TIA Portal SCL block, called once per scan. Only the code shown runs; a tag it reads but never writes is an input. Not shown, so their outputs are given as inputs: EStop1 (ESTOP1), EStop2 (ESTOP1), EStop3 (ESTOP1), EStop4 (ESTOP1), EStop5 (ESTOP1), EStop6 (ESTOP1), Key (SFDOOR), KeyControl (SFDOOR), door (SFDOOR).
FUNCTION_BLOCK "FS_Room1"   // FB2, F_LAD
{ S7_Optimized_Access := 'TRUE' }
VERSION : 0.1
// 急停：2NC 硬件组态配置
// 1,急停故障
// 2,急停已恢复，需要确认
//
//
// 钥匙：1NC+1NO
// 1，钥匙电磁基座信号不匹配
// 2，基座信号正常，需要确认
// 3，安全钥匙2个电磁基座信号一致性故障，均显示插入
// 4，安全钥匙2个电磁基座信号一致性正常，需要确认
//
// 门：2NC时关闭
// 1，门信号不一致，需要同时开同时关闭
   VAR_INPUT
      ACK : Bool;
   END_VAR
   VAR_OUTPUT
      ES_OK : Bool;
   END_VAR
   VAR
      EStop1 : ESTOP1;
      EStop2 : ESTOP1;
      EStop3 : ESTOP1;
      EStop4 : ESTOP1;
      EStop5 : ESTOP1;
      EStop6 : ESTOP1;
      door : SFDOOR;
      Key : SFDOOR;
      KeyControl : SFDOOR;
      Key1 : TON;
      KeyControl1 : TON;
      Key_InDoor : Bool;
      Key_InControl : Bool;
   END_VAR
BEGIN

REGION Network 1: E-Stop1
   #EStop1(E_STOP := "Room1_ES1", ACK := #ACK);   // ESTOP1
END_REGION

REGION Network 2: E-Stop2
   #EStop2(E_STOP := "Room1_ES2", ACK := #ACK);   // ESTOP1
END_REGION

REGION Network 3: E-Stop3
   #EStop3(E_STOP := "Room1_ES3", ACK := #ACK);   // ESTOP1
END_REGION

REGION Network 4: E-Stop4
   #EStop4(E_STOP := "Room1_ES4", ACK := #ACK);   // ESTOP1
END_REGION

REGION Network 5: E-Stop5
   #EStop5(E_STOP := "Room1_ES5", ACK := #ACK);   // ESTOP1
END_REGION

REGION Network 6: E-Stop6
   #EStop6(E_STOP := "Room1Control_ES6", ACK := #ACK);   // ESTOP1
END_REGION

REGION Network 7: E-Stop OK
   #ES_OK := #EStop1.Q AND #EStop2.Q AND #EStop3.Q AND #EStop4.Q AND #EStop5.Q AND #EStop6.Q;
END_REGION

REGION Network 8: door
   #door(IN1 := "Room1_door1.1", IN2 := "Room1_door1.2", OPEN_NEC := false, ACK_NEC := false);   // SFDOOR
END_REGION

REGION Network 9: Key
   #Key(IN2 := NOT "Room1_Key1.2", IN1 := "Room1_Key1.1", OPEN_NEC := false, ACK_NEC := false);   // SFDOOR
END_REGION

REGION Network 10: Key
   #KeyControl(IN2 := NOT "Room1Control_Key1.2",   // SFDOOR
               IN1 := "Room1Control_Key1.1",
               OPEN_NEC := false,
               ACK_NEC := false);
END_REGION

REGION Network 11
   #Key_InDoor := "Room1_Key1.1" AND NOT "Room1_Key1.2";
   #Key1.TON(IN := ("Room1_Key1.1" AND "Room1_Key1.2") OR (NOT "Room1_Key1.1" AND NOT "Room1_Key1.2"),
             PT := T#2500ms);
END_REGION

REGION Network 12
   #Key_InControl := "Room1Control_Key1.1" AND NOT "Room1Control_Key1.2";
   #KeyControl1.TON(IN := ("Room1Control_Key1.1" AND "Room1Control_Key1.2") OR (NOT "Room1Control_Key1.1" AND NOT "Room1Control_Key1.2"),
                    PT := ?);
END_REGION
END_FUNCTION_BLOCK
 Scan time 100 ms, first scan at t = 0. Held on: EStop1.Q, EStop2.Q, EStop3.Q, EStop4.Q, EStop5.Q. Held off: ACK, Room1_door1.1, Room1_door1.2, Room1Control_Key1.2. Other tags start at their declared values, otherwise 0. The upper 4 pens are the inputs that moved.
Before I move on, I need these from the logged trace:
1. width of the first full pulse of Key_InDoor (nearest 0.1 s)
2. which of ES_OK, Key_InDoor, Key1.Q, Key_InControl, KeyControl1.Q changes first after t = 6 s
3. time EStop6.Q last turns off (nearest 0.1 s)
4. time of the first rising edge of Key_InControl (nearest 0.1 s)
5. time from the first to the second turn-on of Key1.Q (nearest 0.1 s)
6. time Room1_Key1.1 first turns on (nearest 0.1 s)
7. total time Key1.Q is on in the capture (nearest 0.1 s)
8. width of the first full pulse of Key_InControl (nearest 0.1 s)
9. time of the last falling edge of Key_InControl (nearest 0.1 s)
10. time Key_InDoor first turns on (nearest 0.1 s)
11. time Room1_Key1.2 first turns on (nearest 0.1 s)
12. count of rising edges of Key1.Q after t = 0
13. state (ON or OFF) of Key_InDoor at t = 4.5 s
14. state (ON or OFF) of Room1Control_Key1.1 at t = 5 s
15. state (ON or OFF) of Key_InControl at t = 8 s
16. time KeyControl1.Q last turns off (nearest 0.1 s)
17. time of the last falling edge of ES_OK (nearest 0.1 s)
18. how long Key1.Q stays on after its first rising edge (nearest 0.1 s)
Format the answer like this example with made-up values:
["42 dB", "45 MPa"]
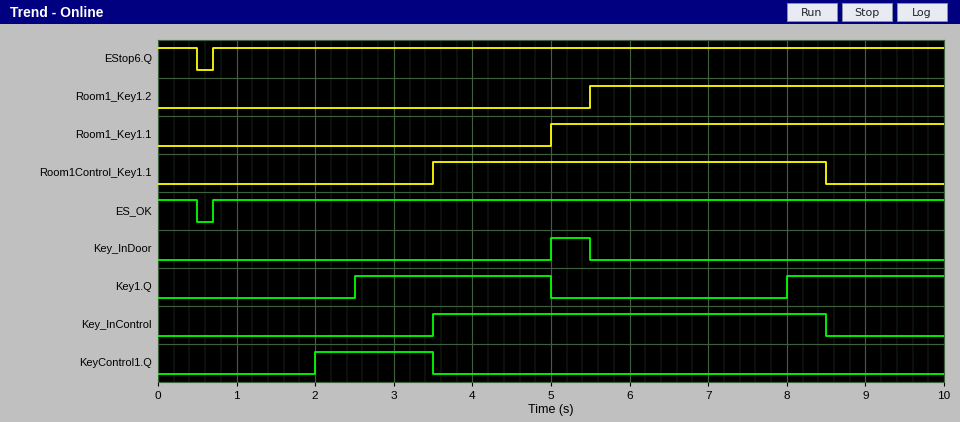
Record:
["0.5 s", "Key1.Q", "0.5 s", "3.5 s", "5.5 s", "5.0 s", "4.5 s", "5.0 s", "8.5 s", "5.0 s", "5.5 s", "2", "OFF", "ON", "ON", "3.5 s", "0.5 s", "2.5 s"]
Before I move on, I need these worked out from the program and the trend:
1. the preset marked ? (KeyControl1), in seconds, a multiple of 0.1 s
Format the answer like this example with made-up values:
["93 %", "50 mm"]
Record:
["2.0 s"]
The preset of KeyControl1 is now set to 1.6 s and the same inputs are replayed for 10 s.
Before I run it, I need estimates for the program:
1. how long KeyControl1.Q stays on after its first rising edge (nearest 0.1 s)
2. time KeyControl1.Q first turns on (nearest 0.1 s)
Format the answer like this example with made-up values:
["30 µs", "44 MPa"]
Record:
["1.9 s", "1.6 s"]
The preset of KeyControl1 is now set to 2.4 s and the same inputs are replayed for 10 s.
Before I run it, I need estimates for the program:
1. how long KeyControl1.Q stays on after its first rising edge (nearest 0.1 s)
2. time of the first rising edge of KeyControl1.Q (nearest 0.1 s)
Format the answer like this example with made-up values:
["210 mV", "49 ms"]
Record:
["1.1 s", "2.4 s"]
